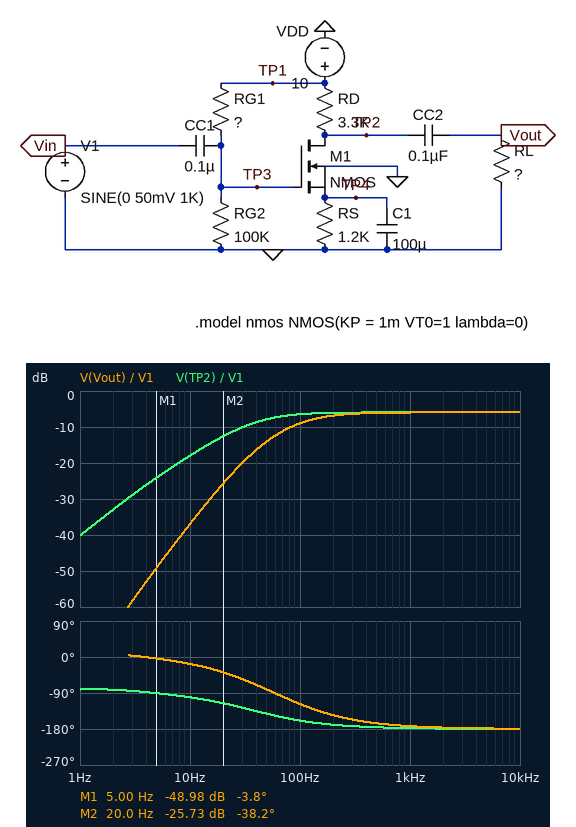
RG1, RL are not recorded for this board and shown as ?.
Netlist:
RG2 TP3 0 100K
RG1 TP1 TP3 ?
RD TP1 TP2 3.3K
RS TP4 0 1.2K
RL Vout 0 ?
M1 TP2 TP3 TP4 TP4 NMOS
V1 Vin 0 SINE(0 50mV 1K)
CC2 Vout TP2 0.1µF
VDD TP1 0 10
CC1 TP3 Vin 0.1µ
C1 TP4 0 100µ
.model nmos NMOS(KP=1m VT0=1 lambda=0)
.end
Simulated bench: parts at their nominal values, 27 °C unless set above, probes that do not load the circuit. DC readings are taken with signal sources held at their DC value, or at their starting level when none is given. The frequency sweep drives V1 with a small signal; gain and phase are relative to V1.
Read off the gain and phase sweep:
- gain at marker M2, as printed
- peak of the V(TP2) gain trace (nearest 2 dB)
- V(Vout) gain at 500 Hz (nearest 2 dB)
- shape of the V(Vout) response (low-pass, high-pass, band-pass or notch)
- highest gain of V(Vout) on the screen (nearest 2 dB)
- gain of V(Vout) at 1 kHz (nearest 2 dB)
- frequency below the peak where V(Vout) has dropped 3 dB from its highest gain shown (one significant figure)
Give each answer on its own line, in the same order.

-25.73 dB
-6 dB
-6 dB
high-pass
-6 dB
-6 dB
100 Hz
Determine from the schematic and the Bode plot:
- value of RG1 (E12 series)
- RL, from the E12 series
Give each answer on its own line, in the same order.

68 kΩ
18 kΩ
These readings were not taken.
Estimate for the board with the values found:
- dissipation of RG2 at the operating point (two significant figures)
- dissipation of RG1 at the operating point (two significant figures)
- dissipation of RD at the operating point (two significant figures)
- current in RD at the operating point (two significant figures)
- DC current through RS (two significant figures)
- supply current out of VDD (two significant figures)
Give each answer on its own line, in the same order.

350 µW
240 µW
13 mW
2.0 mA
2.0 mA
2.1 mA
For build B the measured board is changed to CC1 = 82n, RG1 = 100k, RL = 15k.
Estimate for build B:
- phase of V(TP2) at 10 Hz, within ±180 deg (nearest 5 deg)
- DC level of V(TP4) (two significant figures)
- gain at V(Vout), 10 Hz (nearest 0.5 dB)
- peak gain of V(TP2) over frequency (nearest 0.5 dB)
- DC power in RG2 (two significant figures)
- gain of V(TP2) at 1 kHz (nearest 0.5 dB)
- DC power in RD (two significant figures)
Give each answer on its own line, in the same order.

-90 deg
2.1 V
-17.5 dB
14.5 dB
250 µW
14.0 dB
10 mW
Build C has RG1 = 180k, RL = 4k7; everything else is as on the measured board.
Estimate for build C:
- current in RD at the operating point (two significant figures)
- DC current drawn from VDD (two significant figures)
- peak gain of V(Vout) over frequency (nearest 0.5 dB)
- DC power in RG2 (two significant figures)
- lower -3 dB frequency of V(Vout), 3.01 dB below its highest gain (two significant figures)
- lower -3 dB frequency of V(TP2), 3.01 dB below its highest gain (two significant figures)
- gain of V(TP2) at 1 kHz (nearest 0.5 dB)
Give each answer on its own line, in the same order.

980 µA
1.0 mA
8.5 dB
130 µW
200 Hz
21 Hz
9.0 dB
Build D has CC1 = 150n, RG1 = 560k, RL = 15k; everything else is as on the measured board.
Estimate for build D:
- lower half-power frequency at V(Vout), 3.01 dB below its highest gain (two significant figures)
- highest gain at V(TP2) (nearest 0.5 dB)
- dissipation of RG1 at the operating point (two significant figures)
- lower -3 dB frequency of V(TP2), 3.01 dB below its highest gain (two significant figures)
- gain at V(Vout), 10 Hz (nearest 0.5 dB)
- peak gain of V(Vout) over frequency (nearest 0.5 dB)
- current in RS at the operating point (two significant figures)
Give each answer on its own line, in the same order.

89 Hz
2.0 dB
130 µW
11 Hz
-22.0 dB
1.0 dB
85 µA
